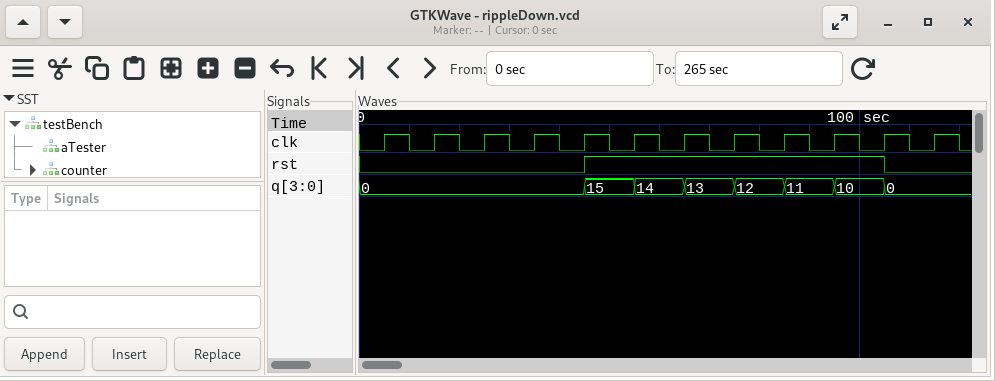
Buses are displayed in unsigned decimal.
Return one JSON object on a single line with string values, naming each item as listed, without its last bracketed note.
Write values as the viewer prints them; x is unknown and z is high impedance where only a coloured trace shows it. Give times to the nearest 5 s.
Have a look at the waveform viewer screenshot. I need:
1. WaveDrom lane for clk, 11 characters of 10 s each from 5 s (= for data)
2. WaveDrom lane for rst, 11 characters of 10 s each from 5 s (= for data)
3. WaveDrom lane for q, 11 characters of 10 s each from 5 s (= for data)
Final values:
{"WaveDrom lane for clk, 11 characters of 10 s each from 5 s": "{name: 'clk', wave: 'p..........'}", "WaveDrom lane for rst, 11 characters of 10 s each from 5 s": "{name: 'rst', wave: '0...1.....0'}", "WaveDrom lane for q, 11 characters of 10 s each from 5 s": "{name: 'q', wave: '=...=======', data: '0 15 14 13 12 11 10 0'}"}
